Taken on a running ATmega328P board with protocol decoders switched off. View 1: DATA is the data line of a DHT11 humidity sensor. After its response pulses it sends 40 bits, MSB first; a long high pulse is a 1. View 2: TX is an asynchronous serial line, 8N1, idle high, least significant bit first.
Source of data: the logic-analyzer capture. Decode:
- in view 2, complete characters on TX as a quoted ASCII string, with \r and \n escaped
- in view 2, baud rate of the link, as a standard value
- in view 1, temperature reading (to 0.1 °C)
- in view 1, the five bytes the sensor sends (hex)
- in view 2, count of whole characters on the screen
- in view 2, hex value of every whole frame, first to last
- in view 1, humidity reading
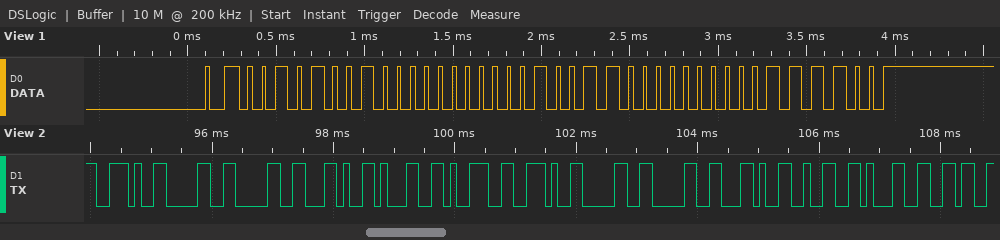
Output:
".00,19.00,216"
9600 baud
19.0 °C
29 00 13 00 3C
13
2E 30 30 2C 31 39 2E 30 30 2C 32 31 36
41 %
